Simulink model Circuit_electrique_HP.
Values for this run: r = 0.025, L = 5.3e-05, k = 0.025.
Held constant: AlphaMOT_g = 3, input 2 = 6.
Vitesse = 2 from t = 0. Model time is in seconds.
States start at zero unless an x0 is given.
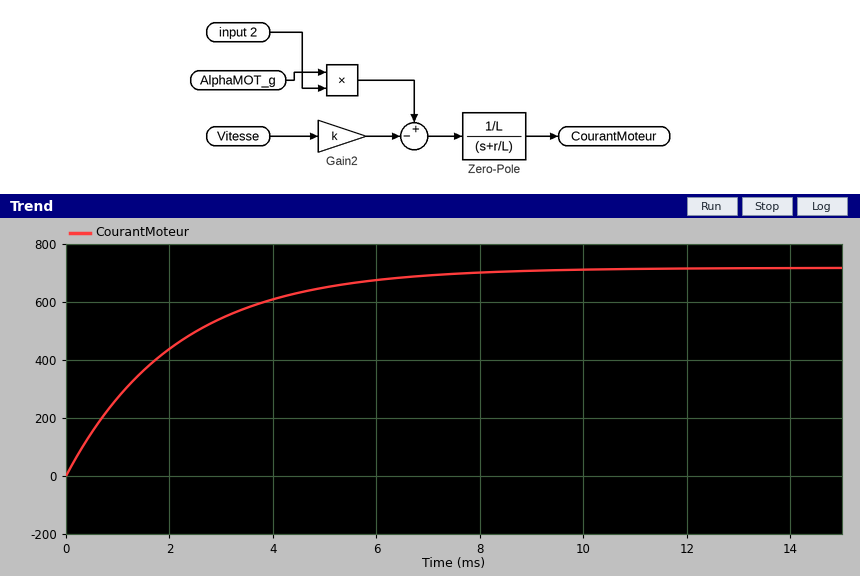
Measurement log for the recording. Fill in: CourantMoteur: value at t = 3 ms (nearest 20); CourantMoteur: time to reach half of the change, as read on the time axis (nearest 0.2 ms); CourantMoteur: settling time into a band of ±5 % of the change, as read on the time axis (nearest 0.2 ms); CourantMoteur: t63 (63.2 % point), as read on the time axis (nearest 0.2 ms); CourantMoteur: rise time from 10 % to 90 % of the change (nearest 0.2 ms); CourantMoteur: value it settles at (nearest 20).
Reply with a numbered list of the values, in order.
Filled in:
1. 540
2. 1.4 ms
3. 6.4 ms
4. 2.2 ms
5. 4.6 ms
6. 720
